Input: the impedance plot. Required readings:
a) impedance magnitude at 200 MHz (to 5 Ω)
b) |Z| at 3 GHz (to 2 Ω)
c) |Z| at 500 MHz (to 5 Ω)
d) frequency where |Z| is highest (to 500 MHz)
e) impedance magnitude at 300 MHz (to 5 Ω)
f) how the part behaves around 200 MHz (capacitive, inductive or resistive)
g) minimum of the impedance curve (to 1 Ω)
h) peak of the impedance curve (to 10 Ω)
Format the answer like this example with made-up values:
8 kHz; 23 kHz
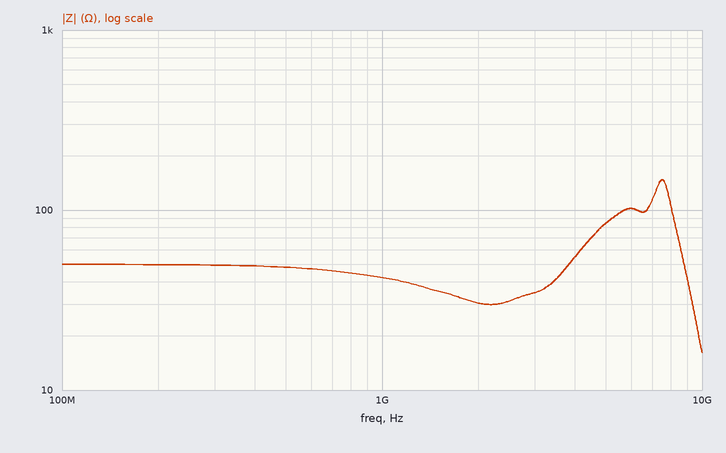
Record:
50 Ω; 34 Ω; 50 Ω; 7.5 GHz; 50 Ω; resistive; 16 Ω; 150 Ω
